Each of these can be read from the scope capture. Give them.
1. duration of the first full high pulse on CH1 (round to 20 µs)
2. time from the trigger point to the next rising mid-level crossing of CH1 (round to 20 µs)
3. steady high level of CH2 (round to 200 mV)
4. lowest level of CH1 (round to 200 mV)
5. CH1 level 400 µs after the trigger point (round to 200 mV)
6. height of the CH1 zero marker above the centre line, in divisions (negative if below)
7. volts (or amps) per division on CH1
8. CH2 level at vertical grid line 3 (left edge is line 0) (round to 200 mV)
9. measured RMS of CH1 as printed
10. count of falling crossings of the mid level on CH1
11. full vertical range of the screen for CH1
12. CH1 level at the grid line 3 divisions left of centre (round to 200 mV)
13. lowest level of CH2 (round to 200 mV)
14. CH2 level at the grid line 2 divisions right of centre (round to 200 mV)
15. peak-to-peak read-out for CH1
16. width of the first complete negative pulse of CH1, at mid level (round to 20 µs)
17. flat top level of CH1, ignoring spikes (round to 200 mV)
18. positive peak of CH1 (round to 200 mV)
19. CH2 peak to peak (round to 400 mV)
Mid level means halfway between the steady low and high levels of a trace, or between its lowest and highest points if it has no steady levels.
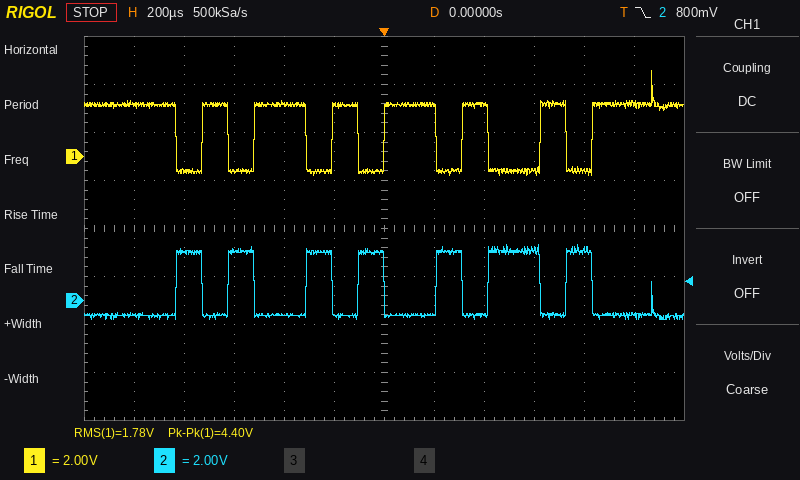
100 µs
320 µs
2.0 V
-800 mV
2.2 V
+1.5 div
2 V
2.0 V
1.78 V
7
16 V
-600 mV
-800 mV
-600 mV
4.40 V
100 µs
2.2 V
3.6 V
3.2 V
